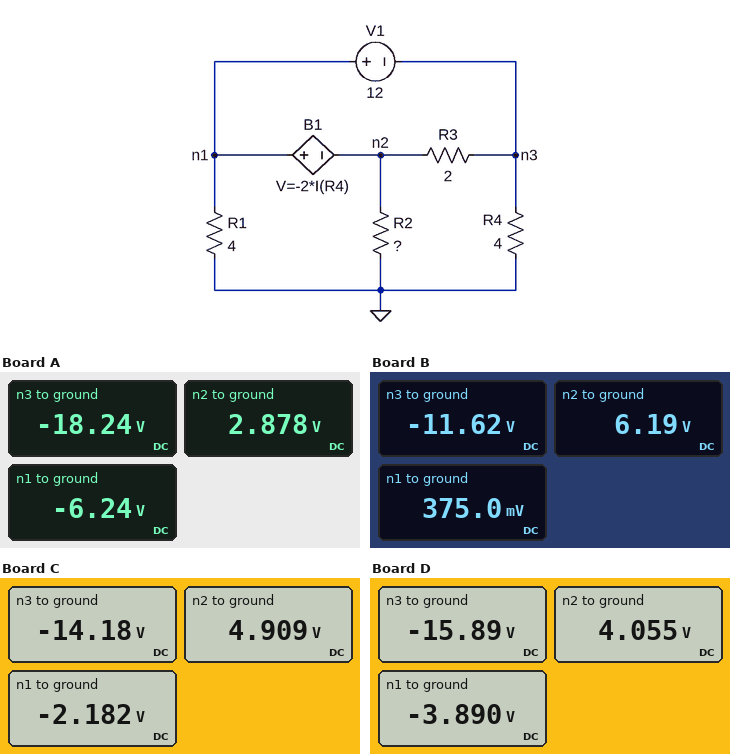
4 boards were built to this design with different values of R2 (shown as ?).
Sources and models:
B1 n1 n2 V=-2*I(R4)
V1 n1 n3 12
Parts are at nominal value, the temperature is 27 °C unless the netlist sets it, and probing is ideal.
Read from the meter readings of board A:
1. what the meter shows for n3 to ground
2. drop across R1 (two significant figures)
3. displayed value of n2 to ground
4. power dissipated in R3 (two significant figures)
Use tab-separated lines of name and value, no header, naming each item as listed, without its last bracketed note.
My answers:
what the meter shows for n3 to ground	-18.24 V
drop across R1	6.2 V
displayed value of n2 to ground	2.878 V
power dissipated in R3	220 W
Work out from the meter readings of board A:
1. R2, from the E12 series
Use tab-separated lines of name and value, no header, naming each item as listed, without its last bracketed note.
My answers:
R2, from the E12 series	0.47 Ω
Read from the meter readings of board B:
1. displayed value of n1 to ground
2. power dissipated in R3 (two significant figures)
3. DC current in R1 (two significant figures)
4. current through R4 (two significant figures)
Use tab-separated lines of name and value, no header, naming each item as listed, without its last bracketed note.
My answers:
displayed value of n1 to ground	375.0 mV
power dissipated in R3	160 W
DC current in R1	94 mA
current through R4	2.9 A
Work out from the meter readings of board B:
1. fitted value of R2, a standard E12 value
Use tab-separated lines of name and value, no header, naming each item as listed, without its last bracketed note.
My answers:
fitted value of R2, a standard E12 value	2.2 Ω
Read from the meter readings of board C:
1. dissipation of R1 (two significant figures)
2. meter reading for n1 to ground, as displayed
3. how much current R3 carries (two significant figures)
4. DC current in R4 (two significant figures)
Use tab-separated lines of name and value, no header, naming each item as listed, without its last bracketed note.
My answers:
dissipation of R1	1.2 W
meter reading for n1 to ground, as displayed	-2.182 V
how much current R3 carries	9.5 A
DC current in R4	3.5 A
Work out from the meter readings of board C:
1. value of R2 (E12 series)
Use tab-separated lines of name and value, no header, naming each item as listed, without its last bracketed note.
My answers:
value of R2	1.2 Ω
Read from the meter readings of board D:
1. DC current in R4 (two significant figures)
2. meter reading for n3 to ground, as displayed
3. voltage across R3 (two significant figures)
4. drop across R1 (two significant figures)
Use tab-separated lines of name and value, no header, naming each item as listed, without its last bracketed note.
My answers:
DC current in R4	4.0 A
meter reading for n3 to ground, as displayed	-15.89 V
voltage across R3	20 V
drop across R1	3.9 V
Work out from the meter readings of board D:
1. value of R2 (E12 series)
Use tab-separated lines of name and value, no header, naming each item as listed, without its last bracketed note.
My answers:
value of R2	0.82 Ω
